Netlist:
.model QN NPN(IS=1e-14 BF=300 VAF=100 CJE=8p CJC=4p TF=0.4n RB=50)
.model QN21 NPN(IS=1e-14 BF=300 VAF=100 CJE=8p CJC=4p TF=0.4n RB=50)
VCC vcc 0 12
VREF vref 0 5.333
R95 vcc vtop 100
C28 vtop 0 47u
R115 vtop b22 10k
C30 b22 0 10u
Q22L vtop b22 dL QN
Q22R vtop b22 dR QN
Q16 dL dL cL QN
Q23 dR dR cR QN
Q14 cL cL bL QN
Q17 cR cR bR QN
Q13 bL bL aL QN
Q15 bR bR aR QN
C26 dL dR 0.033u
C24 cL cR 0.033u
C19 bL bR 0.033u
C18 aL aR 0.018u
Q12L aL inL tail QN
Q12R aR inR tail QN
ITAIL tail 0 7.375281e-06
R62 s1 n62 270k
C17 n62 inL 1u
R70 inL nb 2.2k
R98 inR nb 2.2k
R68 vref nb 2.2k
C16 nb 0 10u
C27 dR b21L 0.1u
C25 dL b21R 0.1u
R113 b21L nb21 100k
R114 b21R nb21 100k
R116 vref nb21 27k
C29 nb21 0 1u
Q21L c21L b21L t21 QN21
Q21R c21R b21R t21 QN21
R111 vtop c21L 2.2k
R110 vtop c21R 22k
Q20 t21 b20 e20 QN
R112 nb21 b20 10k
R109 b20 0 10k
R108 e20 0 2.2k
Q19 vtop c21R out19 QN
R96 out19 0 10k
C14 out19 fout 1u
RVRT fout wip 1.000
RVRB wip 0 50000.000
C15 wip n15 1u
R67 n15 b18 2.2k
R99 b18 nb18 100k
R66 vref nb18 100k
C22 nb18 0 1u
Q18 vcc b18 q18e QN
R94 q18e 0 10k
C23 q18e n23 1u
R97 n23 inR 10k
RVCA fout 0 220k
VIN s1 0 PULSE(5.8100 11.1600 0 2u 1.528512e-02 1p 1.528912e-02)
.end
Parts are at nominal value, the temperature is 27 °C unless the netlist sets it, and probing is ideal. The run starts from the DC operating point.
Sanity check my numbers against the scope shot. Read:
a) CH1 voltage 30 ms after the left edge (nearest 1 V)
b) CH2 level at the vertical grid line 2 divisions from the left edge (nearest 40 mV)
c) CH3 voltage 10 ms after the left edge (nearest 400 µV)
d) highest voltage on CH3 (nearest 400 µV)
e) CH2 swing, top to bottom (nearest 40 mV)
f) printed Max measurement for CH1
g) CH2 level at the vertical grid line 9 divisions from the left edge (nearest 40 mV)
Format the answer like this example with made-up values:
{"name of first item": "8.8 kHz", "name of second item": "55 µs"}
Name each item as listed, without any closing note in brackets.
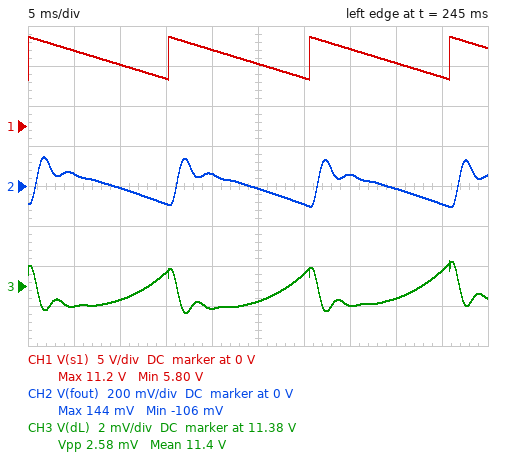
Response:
{"CH1 voltage 30 ms after the left edge": "6 V", "CH2 level at the vertical grid line 2 divisions from the left edge": "0 V", "CH3 voltage 10 ms after the left edge": "11.3752 V", "highest voltage on CH3": "11.3772 V", "CH2 swing, top to bottom": "240 mV", "printed Max measurement for CH1": "11.2 V", "CH2 level at the vertical grid line 9 divisions from the left edge": "-80 mV"}
